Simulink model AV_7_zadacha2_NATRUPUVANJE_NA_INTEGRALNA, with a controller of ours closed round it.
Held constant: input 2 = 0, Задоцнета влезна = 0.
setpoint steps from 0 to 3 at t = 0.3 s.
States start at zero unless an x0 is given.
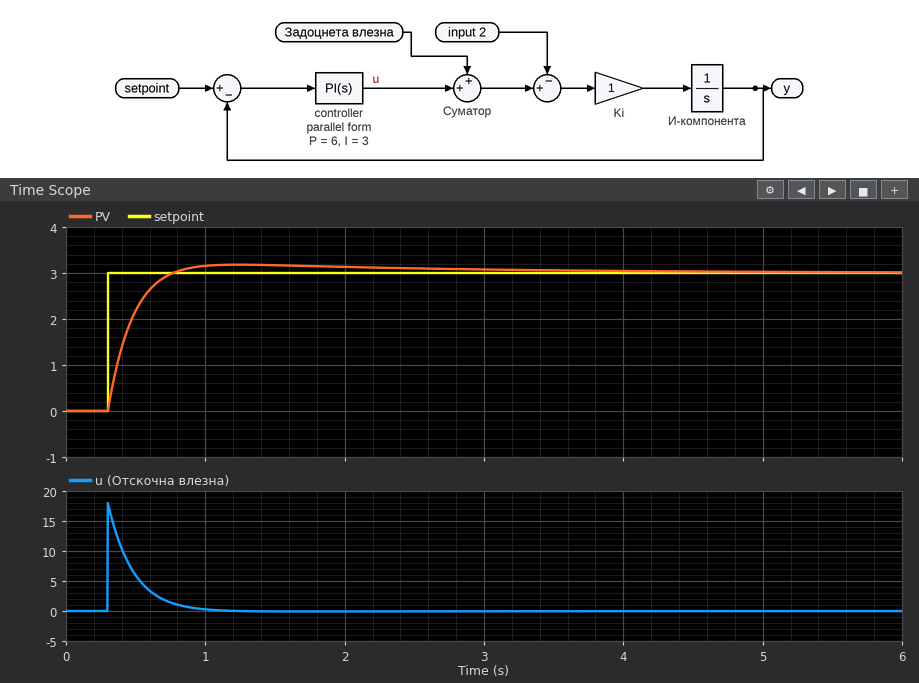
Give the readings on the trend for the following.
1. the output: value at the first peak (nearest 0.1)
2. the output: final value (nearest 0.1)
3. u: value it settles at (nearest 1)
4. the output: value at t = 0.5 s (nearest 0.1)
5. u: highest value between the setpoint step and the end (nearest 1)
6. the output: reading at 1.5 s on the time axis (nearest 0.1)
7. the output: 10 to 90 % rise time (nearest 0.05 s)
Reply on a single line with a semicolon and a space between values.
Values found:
3.2; 3.0; 0; 2.2; 18; 3.2; 0.30 s
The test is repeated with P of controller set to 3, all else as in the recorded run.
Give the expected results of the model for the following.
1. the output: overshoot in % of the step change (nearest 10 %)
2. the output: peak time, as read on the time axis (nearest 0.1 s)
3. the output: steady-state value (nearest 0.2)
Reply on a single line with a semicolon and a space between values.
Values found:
20 %; 1.5 s; 3.0
